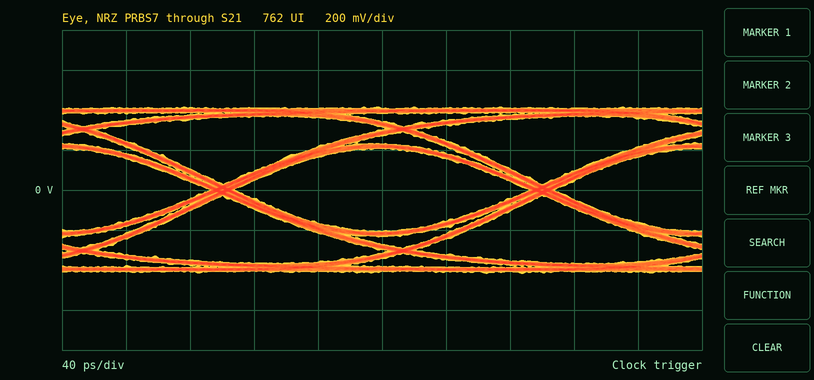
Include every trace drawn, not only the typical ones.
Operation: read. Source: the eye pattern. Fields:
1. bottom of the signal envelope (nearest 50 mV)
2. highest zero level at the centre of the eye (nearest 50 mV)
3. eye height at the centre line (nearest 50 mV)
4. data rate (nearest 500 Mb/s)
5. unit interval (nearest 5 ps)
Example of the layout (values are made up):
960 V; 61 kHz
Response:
-400 mV; -200 mV; 400 mV; 5.0 Gb/s; 200 ps
